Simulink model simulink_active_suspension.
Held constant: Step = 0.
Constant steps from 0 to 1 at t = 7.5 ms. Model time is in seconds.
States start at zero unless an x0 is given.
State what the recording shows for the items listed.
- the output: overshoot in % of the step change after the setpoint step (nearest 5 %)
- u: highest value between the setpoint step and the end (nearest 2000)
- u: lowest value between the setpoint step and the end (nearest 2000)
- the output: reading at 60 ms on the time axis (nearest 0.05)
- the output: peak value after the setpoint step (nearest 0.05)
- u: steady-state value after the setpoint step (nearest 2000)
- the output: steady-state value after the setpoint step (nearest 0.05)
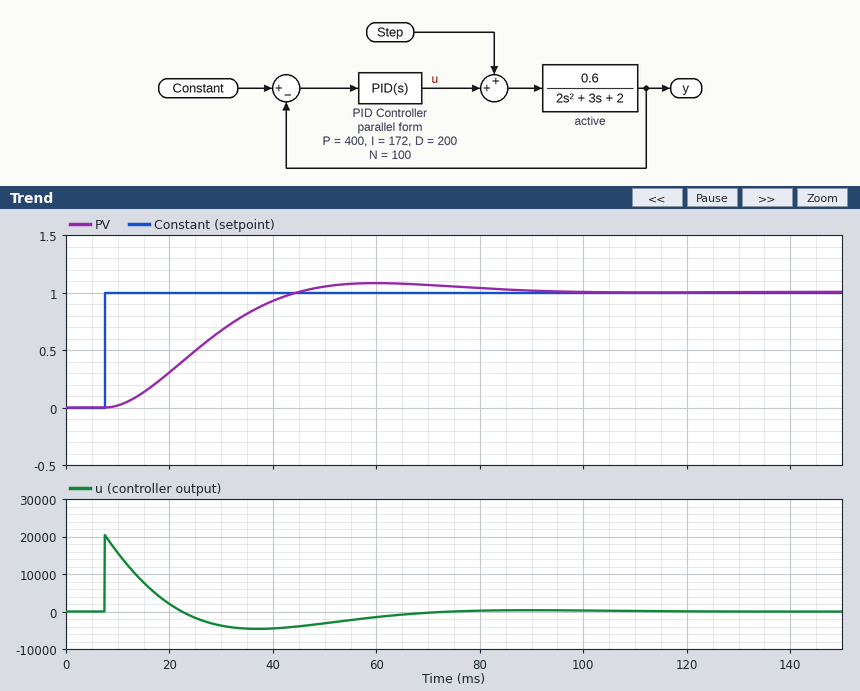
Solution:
10 %
20000
-4000
1.10
1.10
0
1.00
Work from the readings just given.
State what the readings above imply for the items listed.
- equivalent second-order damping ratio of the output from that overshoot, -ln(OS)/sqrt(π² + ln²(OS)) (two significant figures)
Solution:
0.59
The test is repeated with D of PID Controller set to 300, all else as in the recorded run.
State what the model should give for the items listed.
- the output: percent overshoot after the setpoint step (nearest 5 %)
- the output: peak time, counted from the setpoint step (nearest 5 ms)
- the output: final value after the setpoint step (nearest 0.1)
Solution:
15 %
40 ms
1.0
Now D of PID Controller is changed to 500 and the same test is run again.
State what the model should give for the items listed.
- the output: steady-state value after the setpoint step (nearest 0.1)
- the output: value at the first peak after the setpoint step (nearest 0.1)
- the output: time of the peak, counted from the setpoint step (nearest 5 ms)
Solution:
1.0
1.2
30 ms
